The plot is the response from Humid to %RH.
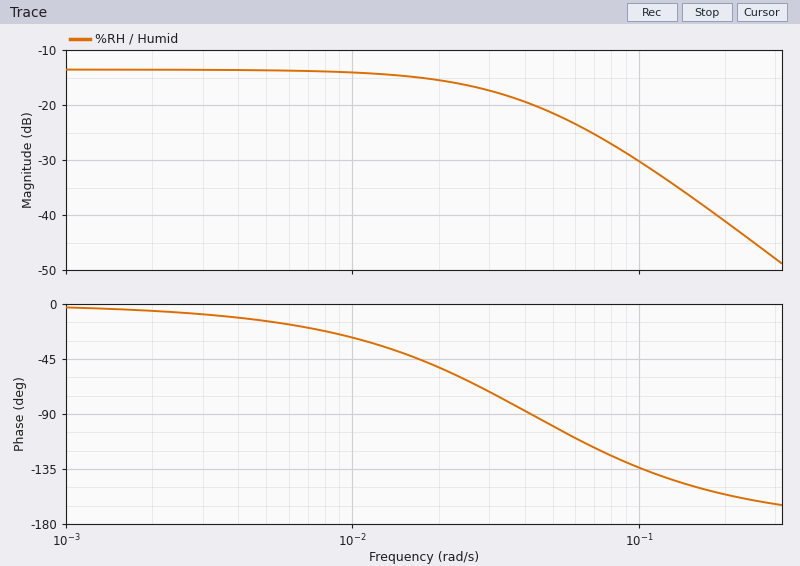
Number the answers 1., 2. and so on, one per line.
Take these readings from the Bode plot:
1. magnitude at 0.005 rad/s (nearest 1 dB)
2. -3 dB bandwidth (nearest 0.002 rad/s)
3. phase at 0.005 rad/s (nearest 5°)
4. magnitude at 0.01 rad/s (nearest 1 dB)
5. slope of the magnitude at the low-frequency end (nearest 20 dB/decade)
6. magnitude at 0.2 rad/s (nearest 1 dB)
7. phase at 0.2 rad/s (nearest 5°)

1. -14 dB
2. 0.026 rad/s
3. -15°
4. -14 dB
5. 0 dB/decade
6. -41 dB
7. -155°
